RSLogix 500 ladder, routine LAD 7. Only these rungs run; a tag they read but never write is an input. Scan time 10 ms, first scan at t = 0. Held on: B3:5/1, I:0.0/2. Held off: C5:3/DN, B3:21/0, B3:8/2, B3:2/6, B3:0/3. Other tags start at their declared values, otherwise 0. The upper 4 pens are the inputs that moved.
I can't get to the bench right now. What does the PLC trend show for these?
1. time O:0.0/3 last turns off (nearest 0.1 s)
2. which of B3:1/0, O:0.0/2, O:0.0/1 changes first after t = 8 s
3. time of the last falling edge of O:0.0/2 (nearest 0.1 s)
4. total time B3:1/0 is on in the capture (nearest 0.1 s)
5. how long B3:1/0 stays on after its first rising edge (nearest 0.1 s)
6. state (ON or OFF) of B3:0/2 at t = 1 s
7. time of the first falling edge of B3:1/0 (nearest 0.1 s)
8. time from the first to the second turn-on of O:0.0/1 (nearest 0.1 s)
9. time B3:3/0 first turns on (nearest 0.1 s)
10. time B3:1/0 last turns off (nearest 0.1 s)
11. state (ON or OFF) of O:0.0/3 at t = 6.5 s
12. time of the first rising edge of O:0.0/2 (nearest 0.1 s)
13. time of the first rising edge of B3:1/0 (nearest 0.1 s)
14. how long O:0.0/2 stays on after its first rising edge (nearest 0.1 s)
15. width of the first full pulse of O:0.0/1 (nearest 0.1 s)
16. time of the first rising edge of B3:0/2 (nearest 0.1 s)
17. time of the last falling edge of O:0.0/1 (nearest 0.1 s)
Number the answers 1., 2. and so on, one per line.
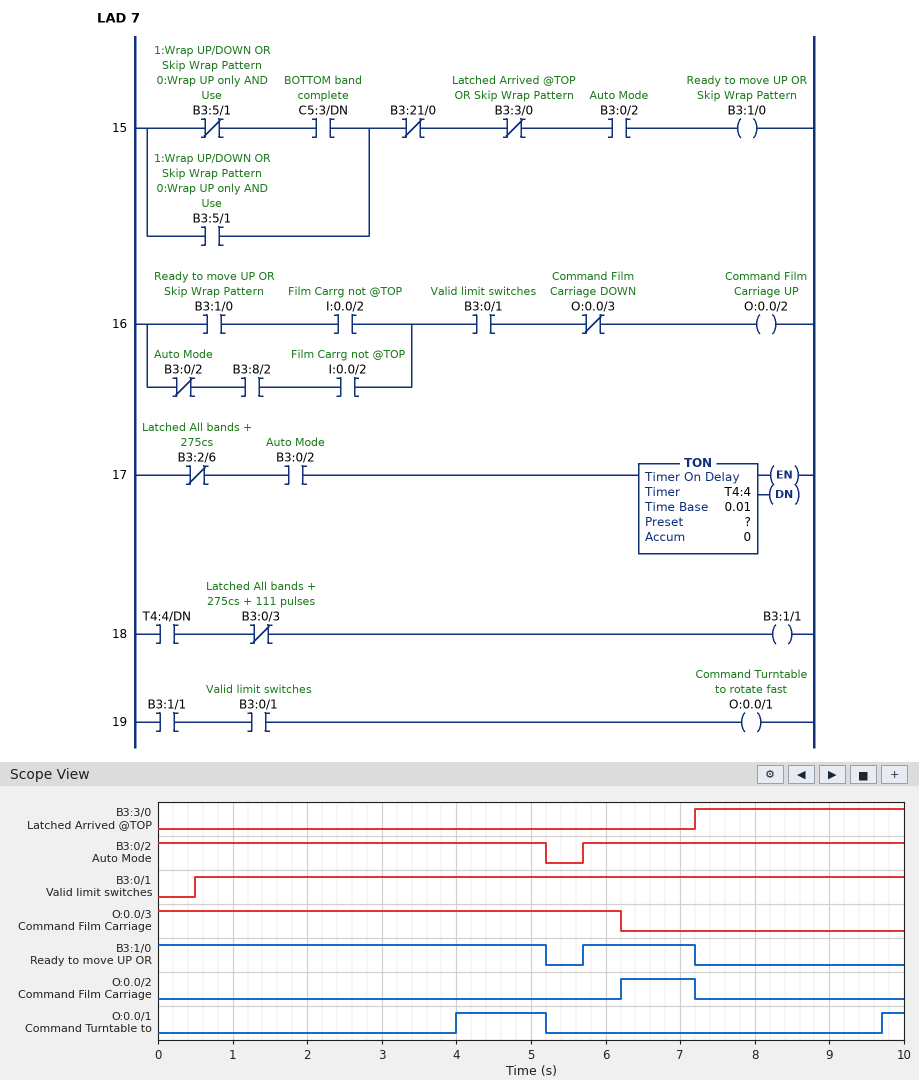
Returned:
1. 6.2 s
2. O:0.0/1
3. 7.2 s
4. 6.7 s
5. 1.5 s
6. ON
7. 5.2 s
8. 5.7 s
9. 7.2 s
10. 7.2 s
11. OFF
12. 6.2 s
13. 5.7 s
14. 1.0 s
15. 1.2 s
16. 5.7 s
17. 5.2 s
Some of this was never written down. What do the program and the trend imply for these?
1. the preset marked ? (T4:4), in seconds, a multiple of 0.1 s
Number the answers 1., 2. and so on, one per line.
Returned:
1. 4.0 s
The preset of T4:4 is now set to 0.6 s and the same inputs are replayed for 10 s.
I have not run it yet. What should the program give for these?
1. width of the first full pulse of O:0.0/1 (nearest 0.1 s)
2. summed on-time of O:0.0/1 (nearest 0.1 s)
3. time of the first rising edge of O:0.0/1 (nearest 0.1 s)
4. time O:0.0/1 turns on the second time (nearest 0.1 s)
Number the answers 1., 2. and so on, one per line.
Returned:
1. 4.6 s
2. 8.3 s
3. 0.6 s
4. 6.3 s
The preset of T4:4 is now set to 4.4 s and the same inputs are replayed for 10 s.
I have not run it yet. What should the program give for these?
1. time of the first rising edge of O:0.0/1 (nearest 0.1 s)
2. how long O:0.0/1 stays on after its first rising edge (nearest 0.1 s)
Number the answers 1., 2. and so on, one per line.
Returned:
1. 4.4 s
2. 0.8 s
